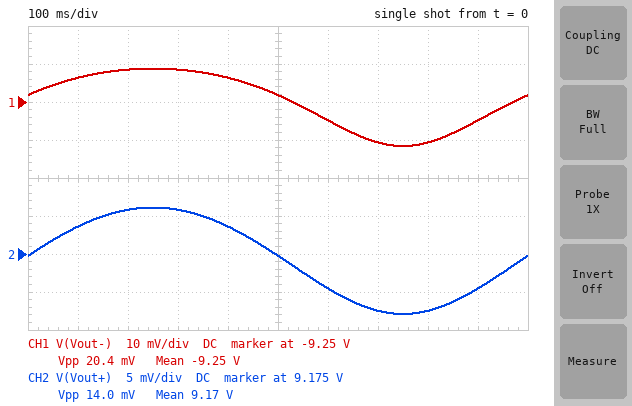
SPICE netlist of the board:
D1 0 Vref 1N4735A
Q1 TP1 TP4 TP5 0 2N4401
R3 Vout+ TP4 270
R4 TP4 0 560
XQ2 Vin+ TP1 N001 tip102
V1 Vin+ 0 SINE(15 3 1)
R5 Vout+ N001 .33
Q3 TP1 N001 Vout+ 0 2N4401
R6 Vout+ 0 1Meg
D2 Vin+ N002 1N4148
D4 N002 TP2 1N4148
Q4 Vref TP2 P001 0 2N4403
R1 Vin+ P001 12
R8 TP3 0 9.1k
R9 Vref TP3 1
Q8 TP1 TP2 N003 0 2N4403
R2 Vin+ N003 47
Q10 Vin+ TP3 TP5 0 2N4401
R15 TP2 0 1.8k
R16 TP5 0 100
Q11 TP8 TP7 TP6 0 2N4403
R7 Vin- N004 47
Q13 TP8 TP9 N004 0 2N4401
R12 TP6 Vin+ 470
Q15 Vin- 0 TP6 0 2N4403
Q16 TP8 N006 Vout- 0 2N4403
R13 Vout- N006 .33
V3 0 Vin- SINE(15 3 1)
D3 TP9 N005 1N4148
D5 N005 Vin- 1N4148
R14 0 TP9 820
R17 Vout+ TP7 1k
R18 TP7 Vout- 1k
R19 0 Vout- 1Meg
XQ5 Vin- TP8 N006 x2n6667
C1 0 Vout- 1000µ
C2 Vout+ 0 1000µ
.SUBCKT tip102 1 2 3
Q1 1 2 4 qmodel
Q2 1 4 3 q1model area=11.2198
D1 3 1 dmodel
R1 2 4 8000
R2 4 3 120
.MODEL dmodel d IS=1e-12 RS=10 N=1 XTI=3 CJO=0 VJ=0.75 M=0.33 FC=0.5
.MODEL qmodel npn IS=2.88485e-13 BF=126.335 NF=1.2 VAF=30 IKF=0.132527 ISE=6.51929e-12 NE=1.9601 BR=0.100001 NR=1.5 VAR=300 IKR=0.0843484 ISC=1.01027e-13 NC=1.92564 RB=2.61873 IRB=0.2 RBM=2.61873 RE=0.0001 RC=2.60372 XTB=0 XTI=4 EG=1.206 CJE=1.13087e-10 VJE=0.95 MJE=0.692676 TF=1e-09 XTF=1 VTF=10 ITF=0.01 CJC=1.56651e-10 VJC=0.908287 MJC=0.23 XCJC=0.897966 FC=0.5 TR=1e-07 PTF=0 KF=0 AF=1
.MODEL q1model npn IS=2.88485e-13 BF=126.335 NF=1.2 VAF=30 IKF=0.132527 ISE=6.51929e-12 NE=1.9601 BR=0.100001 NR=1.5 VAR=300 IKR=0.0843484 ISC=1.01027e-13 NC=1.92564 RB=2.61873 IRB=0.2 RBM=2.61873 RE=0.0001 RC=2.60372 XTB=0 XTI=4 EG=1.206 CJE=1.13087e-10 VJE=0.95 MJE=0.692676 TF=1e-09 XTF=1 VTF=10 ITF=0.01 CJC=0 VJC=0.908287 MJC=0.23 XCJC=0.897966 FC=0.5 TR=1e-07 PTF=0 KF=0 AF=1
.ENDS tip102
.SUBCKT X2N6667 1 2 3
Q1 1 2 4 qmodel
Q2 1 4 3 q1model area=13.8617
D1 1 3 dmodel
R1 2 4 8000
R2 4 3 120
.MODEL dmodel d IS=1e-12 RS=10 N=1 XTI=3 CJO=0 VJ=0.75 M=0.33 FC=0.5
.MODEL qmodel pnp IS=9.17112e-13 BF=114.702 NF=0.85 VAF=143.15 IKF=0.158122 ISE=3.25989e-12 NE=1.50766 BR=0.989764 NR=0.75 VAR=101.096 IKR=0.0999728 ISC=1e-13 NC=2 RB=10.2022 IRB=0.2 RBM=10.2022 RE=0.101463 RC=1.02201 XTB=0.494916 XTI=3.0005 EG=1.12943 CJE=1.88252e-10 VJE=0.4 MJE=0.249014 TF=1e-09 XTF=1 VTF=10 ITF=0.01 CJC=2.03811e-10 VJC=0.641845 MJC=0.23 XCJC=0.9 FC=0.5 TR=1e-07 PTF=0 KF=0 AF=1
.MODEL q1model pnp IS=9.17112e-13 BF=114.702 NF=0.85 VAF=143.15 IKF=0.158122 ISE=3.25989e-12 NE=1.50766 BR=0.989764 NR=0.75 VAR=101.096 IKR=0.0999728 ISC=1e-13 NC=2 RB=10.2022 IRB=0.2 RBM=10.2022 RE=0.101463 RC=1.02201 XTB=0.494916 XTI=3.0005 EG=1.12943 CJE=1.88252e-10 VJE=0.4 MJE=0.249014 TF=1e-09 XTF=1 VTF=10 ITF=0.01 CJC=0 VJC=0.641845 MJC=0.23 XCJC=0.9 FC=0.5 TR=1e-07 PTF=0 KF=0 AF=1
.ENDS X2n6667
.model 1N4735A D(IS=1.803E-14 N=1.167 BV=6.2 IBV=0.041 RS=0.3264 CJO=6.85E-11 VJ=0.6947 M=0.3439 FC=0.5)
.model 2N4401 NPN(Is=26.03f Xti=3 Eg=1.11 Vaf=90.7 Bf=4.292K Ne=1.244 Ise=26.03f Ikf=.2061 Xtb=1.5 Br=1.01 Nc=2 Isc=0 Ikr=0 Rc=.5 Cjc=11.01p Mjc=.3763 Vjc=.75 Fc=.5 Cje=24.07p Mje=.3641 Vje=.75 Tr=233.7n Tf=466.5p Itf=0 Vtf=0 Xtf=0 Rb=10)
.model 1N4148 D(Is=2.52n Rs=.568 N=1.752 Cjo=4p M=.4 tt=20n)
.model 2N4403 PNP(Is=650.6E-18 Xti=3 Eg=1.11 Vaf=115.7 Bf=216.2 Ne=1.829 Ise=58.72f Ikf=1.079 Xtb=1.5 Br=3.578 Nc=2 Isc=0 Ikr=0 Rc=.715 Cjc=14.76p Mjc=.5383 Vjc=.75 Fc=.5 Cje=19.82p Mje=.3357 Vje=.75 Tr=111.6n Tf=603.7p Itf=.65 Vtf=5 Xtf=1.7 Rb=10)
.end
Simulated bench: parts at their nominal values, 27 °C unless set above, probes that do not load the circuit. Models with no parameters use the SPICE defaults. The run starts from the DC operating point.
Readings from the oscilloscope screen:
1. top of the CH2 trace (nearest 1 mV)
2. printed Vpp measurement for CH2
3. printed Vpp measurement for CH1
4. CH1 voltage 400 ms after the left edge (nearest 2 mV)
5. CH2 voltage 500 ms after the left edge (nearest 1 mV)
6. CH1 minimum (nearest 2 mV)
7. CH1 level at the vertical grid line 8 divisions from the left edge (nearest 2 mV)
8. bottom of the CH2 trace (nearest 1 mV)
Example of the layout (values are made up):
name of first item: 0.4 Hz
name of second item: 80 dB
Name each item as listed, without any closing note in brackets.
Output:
top of the CH2 trace: 9.181 V
printed Vpp measurement for CH2: 14.0 mV
printed Vpp measurement for CH1: 20.4 mV
CH1 voltage 400 ms after the left edge: -9.244 V
CH2 voltage 500 ms after the left edge: 9.175 V
CH1 minimum: -9.262 V
CH1 level at the vertical grid line 8 divisions from the left edge: -9.260 V
bottom of the CH2 trace: 9.167 V
